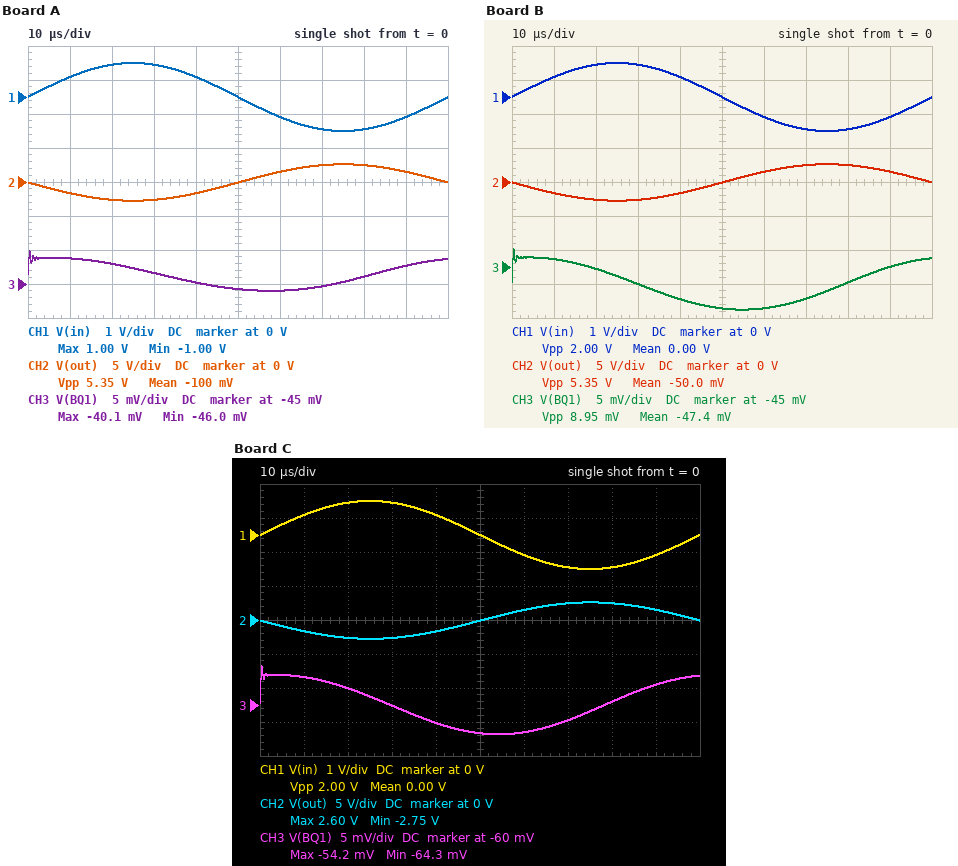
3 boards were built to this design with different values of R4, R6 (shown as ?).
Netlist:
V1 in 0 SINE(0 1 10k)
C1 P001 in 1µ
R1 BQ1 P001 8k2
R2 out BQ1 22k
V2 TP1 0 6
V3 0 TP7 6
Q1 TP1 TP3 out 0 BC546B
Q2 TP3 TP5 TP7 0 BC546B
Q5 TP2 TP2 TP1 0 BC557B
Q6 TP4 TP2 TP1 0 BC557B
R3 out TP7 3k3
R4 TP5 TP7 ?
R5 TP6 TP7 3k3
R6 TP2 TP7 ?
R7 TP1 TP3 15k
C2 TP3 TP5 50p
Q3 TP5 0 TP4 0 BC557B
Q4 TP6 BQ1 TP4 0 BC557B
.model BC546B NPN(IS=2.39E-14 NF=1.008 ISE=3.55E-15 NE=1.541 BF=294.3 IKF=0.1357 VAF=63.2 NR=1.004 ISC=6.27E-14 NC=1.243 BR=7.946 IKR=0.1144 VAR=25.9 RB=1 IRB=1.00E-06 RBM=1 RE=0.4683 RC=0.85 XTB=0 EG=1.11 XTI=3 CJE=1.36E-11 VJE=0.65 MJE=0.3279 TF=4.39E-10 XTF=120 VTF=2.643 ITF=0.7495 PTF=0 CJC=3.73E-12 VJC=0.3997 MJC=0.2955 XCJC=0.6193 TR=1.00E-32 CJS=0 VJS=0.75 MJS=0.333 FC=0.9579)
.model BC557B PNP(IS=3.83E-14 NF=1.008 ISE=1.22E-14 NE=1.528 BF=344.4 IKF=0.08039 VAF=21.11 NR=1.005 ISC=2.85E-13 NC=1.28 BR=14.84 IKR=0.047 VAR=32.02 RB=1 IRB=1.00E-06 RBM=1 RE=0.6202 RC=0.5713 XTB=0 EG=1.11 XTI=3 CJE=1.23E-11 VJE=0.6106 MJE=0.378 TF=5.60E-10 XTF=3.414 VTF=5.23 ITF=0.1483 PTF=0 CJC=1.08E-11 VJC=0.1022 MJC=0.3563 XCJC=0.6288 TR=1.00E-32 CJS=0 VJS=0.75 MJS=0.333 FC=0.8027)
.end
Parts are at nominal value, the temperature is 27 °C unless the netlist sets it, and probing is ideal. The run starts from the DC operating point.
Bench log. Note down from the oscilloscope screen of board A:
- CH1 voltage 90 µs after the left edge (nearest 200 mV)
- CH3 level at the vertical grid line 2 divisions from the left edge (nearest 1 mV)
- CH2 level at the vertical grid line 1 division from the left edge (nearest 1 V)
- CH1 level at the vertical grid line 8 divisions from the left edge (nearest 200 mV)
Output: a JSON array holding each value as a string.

["-600 mV", "-42 mV", "-2 V", "-1.0 V"]
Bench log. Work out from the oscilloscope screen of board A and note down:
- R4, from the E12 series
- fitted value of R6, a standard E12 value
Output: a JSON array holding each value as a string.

["4.7 kΩ", "18 kΩ"]
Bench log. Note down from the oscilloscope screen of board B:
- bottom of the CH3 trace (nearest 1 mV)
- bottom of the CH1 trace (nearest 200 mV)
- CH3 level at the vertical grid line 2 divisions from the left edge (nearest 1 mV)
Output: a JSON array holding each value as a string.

["-51 mV", "-1.0 V", "-45 mV"]
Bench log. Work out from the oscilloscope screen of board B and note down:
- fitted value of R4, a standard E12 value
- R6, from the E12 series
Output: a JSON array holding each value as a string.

["8.2 kΩ", "27 kΩ"]
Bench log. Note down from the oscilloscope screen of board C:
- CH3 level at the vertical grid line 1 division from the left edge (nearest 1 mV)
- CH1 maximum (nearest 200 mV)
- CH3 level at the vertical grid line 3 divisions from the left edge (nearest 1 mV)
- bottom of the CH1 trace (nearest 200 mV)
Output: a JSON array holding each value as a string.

["-56 mV", "1.0 V", "-60 mV", "-1.0 V"]
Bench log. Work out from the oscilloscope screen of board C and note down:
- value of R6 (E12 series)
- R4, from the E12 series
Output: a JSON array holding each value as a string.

["22 kΩ", "10 kΩ"]
